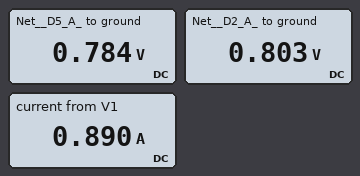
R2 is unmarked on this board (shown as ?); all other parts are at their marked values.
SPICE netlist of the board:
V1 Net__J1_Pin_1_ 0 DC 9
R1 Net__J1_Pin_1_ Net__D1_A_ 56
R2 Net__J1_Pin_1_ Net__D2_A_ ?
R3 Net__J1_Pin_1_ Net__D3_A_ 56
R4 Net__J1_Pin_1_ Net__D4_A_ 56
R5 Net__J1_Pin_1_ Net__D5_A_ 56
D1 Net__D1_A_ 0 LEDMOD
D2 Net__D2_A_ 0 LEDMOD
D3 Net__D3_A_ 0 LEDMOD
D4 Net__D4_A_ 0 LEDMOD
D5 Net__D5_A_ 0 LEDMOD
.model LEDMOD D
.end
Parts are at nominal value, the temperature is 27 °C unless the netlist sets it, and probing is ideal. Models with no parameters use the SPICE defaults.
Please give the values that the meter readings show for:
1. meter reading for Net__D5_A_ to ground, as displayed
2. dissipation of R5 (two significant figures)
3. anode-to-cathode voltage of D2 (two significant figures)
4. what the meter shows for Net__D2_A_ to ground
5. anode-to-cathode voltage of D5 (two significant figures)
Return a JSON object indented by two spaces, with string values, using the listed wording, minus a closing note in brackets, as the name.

{
  "meter reading for Net__D5_A_ to ground, as displayed": "0.784 V",
  "dissipation of R5": "1.2 W",
  "anode-to-cathode voltage of D2": "800 mV",
  "what the meter shows for Net__D2_A_ to ground": "0.803 V",
  "anode-to-cathode voltage of D5": "780 mV"
}
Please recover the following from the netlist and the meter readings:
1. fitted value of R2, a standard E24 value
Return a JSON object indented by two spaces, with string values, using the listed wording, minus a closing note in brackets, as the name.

{
  "fitted value of R2, a standard E24 value": "27 Ω"
}
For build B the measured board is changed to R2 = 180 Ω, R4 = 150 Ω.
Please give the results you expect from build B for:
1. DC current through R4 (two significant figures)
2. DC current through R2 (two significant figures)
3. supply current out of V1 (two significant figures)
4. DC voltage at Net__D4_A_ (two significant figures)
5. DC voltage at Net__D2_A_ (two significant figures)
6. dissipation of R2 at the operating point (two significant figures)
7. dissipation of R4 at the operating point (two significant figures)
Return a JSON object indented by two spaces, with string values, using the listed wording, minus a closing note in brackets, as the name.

{
  "DC current through R4": "55 mA",
  "DC current through R2": "46 mA",
  "supply current out of V1": "540 mA",
  "DC voltage at Net__D4_A_": "760 mV",
  "DC voltage at Net__D2_A_": "750 mV",
  "dissipation of R2 at the operating point": "380 mW",
  "dissipation of R4 at the operating point": "450 mW"
}
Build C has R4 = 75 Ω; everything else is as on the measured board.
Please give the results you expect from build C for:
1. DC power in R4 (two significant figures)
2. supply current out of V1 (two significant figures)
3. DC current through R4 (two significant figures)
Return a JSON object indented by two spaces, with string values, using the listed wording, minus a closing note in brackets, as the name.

{
  "DC power in R4": "900 mW",
  "supply current out of V1": "850 mA",
  "DC current through R4": "110 mA"
}
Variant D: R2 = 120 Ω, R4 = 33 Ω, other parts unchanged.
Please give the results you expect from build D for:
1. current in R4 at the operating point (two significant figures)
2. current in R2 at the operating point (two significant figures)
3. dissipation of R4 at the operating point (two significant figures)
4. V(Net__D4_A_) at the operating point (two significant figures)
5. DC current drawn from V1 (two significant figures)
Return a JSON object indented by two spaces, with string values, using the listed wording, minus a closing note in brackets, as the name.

{
  "current in R4 at the operating point": "250 mA",
  "current in R2 at the operating point": "69 mA",
  "dissipation of R4 at the operating point": "2.0 W",
  "V(Net__D4_A_) at the operating point": "800 mV",
  "DC current drawn from V1": "760 mA"
}
